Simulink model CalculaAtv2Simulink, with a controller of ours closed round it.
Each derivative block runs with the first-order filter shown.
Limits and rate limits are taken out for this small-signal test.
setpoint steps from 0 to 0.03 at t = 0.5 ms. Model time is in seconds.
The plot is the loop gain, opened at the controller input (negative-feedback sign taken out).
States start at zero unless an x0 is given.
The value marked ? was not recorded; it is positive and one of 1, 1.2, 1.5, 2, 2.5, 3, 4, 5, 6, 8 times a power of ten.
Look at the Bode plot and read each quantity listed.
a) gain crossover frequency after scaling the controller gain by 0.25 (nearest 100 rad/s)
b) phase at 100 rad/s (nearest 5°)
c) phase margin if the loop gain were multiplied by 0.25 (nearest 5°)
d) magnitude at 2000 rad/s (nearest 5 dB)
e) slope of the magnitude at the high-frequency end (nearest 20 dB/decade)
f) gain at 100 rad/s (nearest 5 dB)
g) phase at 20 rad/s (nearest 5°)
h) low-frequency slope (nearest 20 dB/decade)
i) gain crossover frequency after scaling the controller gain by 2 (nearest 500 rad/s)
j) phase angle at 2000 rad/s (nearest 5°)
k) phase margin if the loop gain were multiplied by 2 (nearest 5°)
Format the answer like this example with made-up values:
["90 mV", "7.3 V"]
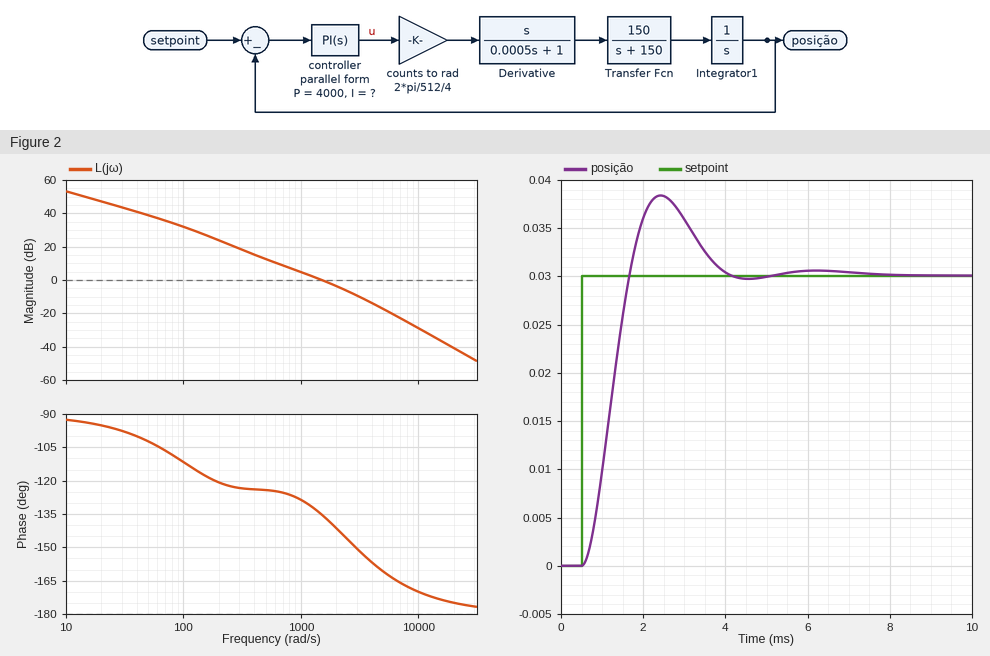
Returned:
["500 rad/s", "-110°", "55°", "-5 dB", "-40 dB/decade", "30 dB", "-95°", "-20 dB/decade", "2500 rad/s", "-140°", "35°"]
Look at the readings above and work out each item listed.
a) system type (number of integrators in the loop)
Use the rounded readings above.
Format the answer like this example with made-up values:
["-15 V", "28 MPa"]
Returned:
["1"]
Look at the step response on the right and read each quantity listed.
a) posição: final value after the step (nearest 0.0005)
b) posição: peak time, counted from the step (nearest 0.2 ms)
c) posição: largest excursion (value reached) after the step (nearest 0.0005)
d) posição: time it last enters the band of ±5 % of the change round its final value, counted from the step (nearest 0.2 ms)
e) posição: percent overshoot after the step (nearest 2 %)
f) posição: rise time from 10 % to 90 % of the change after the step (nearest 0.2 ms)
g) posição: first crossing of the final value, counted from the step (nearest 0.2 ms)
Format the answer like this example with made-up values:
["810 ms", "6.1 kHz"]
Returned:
["0.0300", "2.0 ms", "0.0385", "3.2 ms", "28 %", "0.8 ms", "1.2 ms"]
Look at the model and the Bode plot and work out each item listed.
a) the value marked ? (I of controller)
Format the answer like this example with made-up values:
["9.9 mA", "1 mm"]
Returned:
["1.5e+06"]
